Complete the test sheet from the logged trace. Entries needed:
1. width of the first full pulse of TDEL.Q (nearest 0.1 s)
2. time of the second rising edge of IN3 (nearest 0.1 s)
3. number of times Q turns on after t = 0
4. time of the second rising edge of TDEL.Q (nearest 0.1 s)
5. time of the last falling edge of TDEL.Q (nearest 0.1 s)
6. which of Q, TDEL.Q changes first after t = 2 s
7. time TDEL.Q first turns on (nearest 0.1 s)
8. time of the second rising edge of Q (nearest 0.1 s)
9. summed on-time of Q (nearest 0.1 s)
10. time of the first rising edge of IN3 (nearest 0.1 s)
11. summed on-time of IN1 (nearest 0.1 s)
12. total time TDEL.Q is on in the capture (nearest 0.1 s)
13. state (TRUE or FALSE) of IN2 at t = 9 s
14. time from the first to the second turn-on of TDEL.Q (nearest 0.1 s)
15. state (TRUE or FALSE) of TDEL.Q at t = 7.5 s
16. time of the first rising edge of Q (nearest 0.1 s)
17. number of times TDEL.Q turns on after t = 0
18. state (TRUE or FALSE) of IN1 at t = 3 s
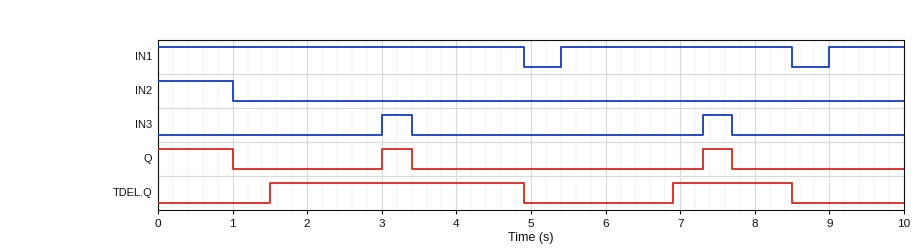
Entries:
3.4 s
7.3 s
2
6.9 s
8.5 s
Q
1.5 s
7.3 s
1.8 s
3.0 s
9.0 s
5.0 s
FALSE
5.4 s
TRUE
3.0 s
2
TRUE
